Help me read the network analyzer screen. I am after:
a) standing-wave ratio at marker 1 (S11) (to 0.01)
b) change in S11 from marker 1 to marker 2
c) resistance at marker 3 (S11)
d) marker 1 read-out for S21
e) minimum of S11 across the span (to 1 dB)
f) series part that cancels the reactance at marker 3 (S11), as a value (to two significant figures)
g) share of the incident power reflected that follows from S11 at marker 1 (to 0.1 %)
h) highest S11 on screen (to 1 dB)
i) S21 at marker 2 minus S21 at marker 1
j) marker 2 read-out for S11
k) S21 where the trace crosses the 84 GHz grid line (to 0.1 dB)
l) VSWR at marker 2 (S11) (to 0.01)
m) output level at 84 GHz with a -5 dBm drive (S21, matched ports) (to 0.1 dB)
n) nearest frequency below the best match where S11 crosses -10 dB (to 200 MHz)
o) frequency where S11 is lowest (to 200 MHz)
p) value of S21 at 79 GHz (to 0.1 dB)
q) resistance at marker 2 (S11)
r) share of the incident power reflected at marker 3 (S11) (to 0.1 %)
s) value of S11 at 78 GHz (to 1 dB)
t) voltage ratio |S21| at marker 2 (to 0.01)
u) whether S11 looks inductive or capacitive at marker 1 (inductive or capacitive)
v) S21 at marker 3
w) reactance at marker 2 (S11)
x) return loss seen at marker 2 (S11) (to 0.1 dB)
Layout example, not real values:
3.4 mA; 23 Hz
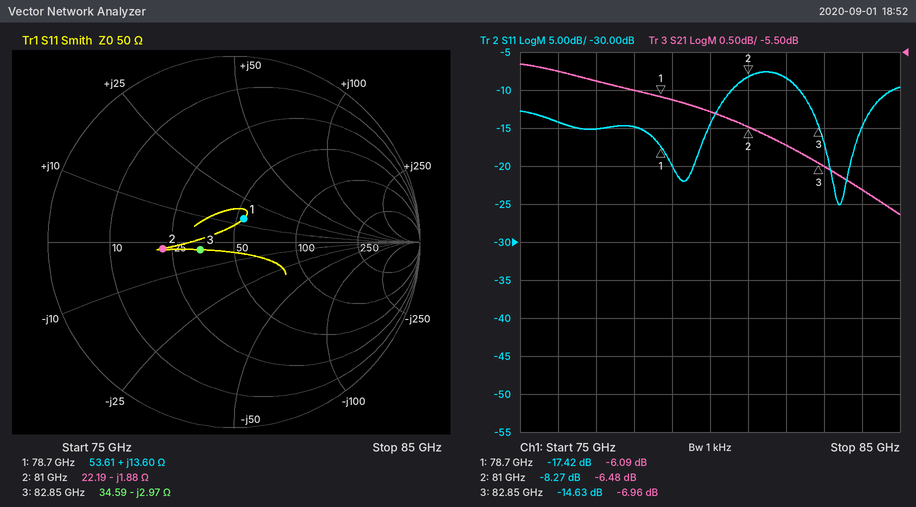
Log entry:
1.31; 9.15 dB; 34.59 Ω; -6.09 dB; -25 dB; 5.7 pH; 1.8 %; -8 dB; -0.39 dB; -8.27 dB; -7.3 dB; 2.26; -12.3 dBm; 82.4 GHz; 83.4 GHz; -6.1 dB; 22.19 Ω; 3.4 %; -15 dB; 0.47; inductive; -6.96 dB; -1.88 Ω; 8.3 dB
